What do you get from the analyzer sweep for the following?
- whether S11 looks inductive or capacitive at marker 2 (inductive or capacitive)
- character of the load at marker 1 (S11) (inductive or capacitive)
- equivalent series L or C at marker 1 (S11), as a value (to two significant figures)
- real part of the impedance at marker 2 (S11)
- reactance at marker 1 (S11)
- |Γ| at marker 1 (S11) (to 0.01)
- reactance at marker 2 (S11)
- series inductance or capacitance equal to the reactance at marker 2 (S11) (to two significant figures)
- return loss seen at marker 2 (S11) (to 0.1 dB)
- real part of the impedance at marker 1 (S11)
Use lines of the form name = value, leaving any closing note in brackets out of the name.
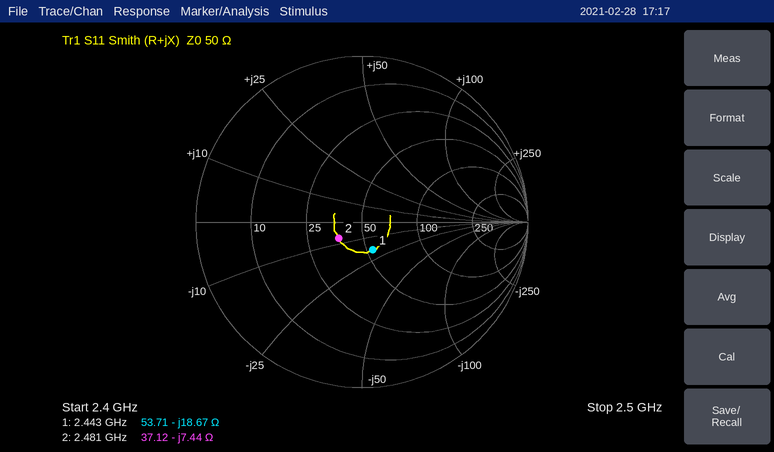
whether S11 looks inductive or capacitive at marker 2 = capacitive
character of the load at marker 1 (S11) = capacitive
equivalent series L or C at marker 1 (S11), as a value = 3.5 pF
real part of the impedance at marker 2 = 37.12 Ω
reactance at marker 1 = -18.67 Ω
|Γ| at marker 1 (S11) = 0.18
reactance at marker 2 = -7.44 Ω
series inductance or capacitance equal to the reactance at marker 2 (S11) = 8.6 pF
return loss seen at marker 2 (S11) = 15.4 dB
real part of the impedance at marker 1 = 53.71 Ω
